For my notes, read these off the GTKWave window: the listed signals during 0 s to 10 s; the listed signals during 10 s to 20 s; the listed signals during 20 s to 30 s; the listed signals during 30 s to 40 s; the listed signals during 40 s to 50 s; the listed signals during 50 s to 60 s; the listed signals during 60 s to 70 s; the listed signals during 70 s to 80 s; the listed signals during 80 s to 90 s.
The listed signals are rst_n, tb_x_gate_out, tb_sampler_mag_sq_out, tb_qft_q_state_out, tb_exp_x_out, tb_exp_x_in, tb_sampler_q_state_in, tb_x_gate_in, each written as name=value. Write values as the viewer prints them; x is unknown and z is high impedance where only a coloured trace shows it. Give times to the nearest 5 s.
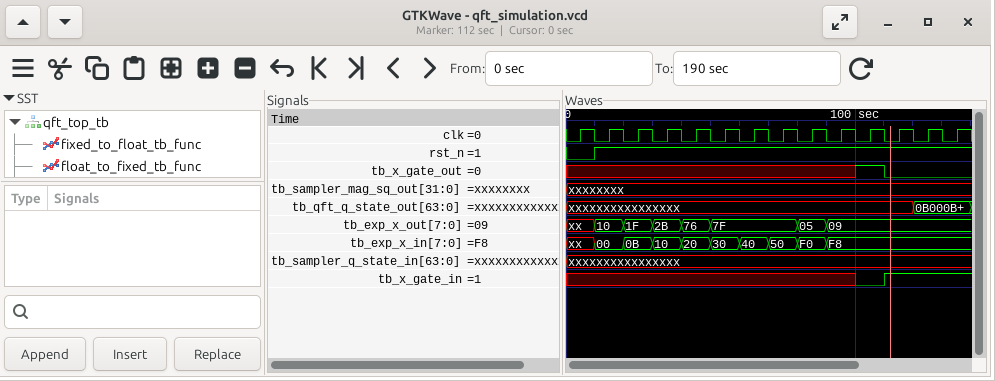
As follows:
rst_n=0, tb_x_gate_out=x, tb_sampler_mag_sq_out=xxxxxxxx, tb_qft_q_state_out=xxxxxxxxxxxxxxxx, tb_exp_x_out=xx, tb_exp_x_in=xx, tb_sampler_q_state_in=xxxxxxxxxxxxxxxx, tb_x_gate_in=x
rst_n=1, tb_x_gate_out=x, tb_sampler_mag_sq_out=xxxxxxxx, tb_qft_q_state_out=xxxxxxxxxxxxxxxx, tb_exp_x_out=10, tb_exp_x_in=00, tb_sampler_q_state_in=xxxxxxxxxxxxxxxx, tb_x_gate_in=x
rst_n=1, tb_x_gate_out=x, tb_sampler_mag_sq_out=xxxxxxxx, tb_qft_q_state_out=xxxxxxxxxxxxxxxx, tb_exp_x_out=1F, tb_exp_x_in=0B, tb_sampler_q_state_in=xxxxxxxxxxxxxxxx, tb_x_gate_in=x
rst_n=1, tb_x_gate_out=x, tb_sampler_mag_sq_out=xxxxxxxx, tb_qft_q_state_out=xxxxxxxxxxxxxxxx, tb_exp_x_out=2B, tb_exp_x_in=10, tb_sampler_q_state_in=xxxxxxxxxxxxxxxx, tb_x_gate_in=x
rst_n=1, tb_x_gate_out=x, tb_sampler_mag_sq_out=xxxxxxxx, tb_qft_q_state_out=xxxxxxxxxxxxxxxx, tb_exp_x_out=76, tb_exp_x_in=20, tb_sampler_q_state_in=xxxxxxxxxxxxxxxx, tb_x_gate_in=x
rst_n=1, tb_x_gate_out=x, tb_sampler_mag_sq_out=xxxxxxxx, tb_qft_q_state_out=xxxxxxxxxxxxxxxx, tb_exp_x_out=7F, tb_exp_x_in=30, tb_sampler_q_state_in=xxxxxxxxxxxxxxxx, tb_x_gate_in=x
rst_n=1, tb_x_gate_out=x, tb_sampler_mag_sq_out=xxxxxxxx, tb_qft_q_state_out=xxxxxxxxxxxxxxxx, tb_exp_x_out=7F, tb_exp_x_in=40, tb_sampler_q_state_in=xxxxxxxxxxxxxxxx, tb_x_gate_in=x
rst_n=1, tb_x_gate_out=x, tb_sampler_mag_sq_out=xxxxxxxx, tb_qft_q_state_out=xxxxxxxxxxxxxxxx, tb_exp_x_out=7F, tb_exp_x_in=50, tb_sampler_q_state_in=xxxxxxxxxxxxxxxx, tb_x_gate_in=x
rst_n=1, tb_x_gate_out=x, tb_sampler_mag_sq_out=xxxxxxxx, tb_qft_q_state_out=xxxxxxxxxxxxxxxx, tb_exp_x_out=05, tb_exp_x_in=F0, tb_sampler_q_state_in=xxxxxxxxxxxxxxxx, tb_x_gate_in=x
